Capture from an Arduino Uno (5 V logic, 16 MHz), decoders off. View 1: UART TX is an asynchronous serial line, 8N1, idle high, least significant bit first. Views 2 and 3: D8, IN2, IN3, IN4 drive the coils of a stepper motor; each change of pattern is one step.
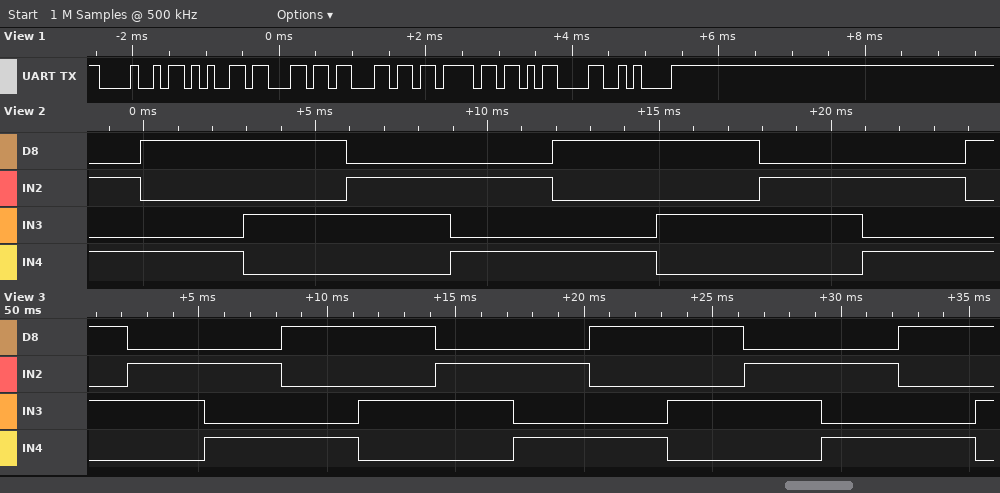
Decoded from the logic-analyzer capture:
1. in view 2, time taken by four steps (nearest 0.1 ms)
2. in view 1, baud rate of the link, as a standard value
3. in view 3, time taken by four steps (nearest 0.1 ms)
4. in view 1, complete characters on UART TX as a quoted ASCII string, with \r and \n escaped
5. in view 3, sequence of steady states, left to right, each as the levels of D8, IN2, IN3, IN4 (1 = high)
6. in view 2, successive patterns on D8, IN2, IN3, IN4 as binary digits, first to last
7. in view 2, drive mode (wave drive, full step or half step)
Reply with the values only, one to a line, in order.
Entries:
12.0 ms
9600 baud
12.0 ms
"Hello\r\n"
1010 0110 0101 1001 1010 0110 0101 1001 1010 0110 0101 1001 1010
0101 1001 1010 0110 0101 1001 1010 0110 0101 1001
full step
